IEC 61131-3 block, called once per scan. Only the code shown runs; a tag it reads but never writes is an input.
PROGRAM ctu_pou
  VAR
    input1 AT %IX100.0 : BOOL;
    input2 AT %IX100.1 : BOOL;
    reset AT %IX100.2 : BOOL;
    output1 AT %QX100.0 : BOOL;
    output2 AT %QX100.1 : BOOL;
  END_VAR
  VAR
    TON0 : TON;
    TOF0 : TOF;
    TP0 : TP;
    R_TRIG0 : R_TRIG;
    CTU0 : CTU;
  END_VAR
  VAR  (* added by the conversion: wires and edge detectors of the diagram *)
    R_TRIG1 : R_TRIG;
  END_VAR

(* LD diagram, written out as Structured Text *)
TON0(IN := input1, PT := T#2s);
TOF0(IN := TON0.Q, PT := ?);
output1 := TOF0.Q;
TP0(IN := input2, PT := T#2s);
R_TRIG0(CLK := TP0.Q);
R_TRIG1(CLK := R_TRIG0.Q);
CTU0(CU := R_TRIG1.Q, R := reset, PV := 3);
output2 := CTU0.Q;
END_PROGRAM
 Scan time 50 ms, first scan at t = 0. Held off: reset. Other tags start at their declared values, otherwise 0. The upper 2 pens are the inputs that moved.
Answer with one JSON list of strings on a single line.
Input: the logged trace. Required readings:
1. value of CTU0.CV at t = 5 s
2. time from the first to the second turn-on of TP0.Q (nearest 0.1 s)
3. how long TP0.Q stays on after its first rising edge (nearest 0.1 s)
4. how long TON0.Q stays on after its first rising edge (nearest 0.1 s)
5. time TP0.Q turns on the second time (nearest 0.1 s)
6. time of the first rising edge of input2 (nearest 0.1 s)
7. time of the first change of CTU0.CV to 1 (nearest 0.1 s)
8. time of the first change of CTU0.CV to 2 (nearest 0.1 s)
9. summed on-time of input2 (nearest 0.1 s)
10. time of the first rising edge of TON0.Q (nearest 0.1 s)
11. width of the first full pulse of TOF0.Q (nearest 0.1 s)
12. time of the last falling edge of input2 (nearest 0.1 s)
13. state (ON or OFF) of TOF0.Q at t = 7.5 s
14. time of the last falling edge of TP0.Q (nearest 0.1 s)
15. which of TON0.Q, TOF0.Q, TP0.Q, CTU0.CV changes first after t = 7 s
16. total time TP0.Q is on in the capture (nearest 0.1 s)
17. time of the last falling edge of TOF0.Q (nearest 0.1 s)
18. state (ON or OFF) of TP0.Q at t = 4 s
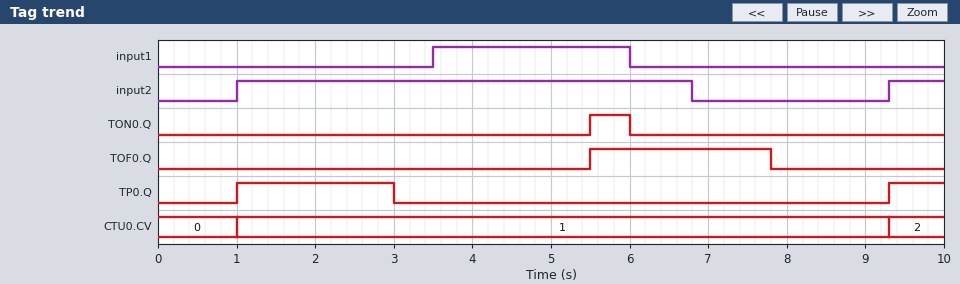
["1", "8.3 s", "2.0 s", "0.5 s", "9.3 s", "1.0 s", "1.0 s", "9.3 s", "6.5 s", "5.5 s", "2.3 s", "6.8 s", "ON", "3.0 s", "TOF0.Q", "2.7 s", "7.8 s", "OFF"]
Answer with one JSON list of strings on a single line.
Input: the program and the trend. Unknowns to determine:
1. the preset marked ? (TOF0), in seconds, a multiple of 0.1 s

["1.8 s"]
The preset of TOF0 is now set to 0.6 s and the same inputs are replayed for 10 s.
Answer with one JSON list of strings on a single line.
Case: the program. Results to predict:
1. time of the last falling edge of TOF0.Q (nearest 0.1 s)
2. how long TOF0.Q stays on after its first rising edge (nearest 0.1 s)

["6.6 s", "1.1 s"]
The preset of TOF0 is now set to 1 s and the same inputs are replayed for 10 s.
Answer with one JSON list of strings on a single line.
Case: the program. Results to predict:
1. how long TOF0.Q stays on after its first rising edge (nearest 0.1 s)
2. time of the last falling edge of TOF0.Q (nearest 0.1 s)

["1.5 s", "7.0 s"]
